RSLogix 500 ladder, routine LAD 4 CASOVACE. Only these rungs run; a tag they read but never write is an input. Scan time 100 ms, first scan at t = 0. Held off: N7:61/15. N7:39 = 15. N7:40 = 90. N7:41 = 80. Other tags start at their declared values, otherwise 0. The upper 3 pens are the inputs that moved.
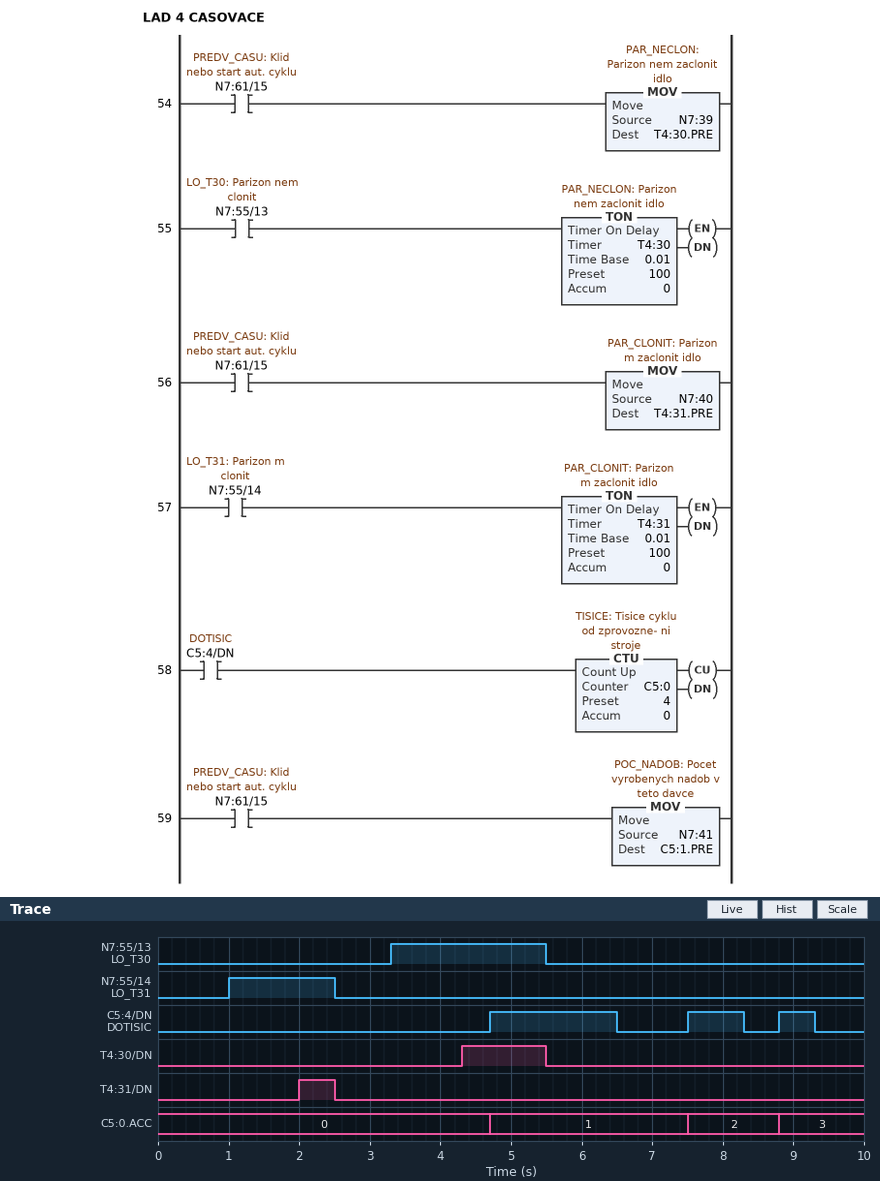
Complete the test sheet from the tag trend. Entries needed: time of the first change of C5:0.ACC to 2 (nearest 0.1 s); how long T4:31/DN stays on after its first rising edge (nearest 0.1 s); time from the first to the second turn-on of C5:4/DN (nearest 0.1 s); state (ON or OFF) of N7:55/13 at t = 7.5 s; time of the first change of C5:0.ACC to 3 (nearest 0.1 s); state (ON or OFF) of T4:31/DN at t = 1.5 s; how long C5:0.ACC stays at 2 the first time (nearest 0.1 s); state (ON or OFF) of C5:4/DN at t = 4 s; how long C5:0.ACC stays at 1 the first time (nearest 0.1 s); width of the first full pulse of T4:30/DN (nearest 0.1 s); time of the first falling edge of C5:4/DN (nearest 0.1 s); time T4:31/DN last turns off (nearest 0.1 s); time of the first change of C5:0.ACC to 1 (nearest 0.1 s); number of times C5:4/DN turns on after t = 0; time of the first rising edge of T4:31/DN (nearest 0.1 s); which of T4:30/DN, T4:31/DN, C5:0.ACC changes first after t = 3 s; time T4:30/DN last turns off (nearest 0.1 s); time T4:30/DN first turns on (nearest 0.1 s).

7.5 s
0.5 s
2.8 s
OFF
8.8 s
OFF
1.3 s
OFF
2.8 s
1.2 s
6.5 s
2.5 s
4.7 s
3
2.0 s
T4:30/DN
5.5 s
4.3 s
